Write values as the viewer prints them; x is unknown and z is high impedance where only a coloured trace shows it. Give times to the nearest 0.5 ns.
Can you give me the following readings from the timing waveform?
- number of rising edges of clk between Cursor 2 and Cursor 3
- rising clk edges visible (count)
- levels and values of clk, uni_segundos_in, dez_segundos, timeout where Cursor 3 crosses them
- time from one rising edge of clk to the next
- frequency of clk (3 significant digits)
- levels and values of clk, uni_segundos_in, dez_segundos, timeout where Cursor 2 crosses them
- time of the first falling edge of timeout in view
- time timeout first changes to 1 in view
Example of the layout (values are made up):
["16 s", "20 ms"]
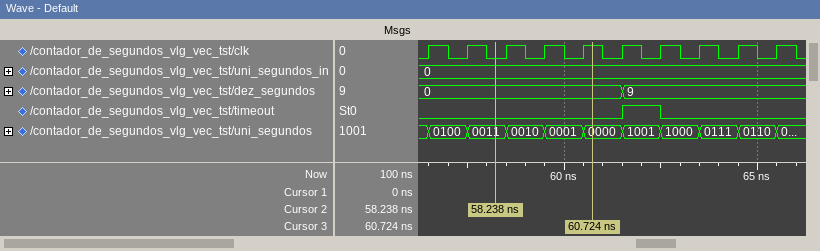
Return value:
["3", "10", "clk=1, uni_segundos_in=0, dez_segundos=0, timeout=0", "1 ns", "1.00 GHz", "clk=0, uni_segundos_in=0, dez_segundos=0, timeout=0", "62.5 ns", "61.5 ns"]
